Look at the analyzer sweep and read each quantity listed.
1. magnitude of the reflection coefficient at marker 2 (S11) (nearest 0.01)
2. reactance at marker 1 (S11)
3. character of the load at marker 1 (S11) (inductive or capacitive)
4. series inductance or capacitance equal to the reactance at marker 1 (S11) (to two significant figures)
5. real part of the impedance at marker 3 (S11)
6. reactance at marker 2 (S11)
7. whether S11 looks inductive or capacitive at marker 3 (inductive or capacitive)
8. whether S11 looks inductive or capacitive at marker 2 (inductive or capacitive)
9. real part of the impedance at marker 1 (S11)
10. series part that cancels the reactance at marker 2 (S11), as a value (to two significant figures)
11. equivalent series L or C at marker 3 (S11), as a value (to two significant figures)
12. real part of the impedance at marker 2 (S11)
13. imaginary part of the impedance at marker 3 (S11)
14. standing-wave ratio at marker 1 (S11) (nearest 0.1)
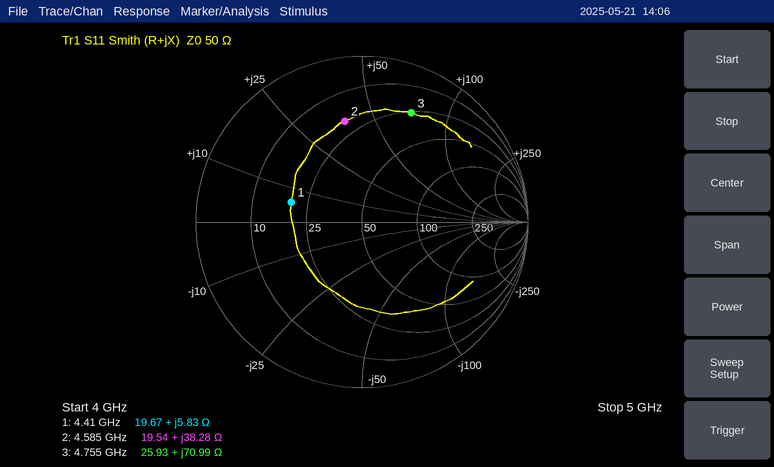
0.62
+5.83 Ω
inductive
210 pH
25.93 Ω
+38.28 Ω
inductive
inductive
19.67 Ω
910 fF
2.4 nH
19.54 Ω
+70.99 Ω
2.6
